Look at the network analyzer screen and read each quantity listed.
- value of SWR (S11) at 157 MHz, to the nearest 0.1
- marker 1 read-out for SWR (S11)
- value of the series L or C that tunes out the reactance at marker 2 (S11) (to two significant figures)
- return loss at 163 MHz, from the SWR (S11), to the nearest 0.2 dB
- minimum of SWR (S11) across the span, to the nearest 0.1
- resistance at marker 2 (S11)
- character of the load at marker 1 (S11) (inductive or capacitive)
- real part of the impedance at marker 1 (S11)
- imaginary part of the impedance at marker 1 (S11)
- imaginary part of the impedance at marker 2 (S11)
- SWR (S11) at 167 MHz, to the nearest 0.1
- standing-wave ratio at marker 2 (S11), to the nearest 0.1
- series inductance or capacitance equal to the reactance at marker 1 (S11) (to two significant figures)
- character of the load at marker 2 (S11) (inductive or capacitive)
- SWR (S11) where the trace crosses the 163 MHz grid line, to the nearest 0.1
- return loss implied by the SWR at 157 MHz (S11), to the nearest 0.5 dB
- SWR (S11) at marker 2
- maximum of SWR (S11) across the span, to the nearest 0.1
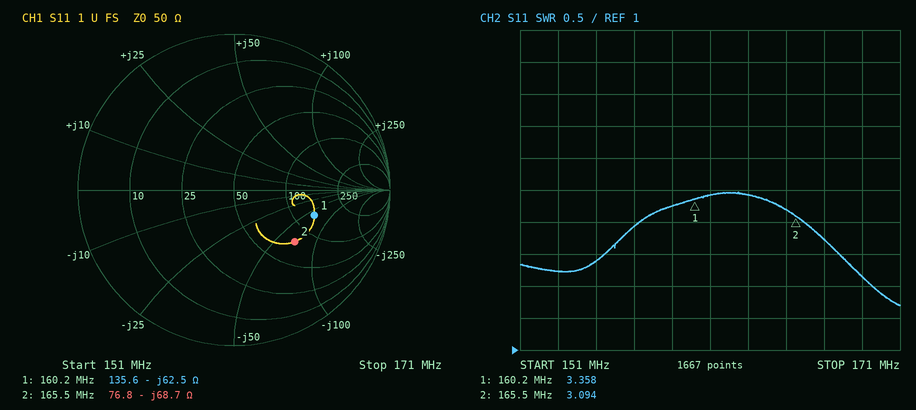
2.9
3.358
66 nH
5.2 dB
1.7
76.8 Ω
capacitive
135.6 Ω
-62.5 Ω
-68.7 Ω
2.7
3.1
16 pF
capacitive
3.4
6.0 dB
3.094
3.5
